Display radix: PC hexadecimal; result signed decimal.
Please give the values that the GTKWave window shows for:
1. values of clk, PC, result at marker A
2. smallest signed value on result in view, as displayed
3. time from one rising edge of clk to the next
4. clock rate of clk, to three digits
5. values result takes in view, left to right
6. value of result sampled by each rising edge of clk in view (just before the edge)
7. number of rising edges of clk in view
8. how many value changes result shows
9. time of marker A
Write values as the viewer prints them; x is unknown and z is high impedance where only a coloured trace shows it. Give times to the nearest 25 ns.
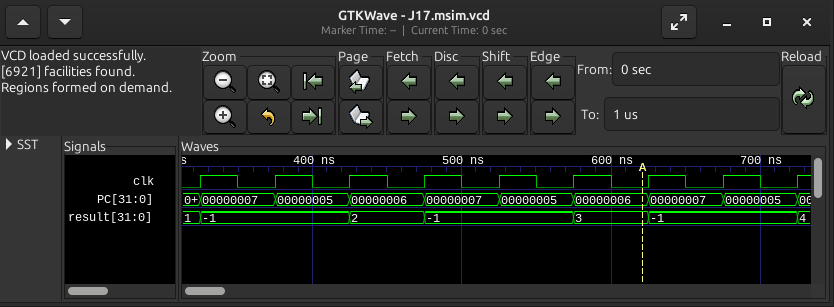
clk=0, PC=00000006, result=3
-1
50 ns
20.0 MHz
1, -1, 2, -1, 3, -1, 4
1, -1, -1, 2, -1, -1, 3, -1, -1
9
6
625 ns
